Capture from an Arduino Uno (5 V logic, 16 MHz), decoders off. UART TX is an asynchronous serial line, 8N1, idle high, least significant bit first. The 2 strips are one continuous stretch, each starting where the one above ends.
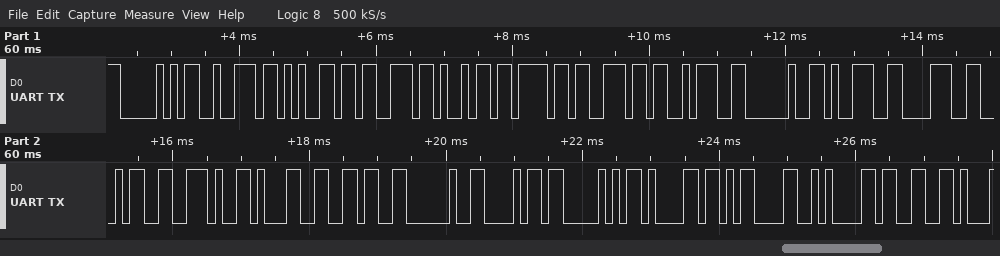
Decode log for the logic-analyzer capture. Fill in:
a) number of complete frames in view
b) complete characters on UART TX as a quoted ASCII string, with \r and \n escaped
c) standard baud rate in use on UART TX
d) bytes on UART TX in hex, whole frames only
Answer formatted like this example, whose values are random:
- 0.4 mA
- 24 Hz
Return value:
- 22
- "Presion: 984.16 hPa\r\n3"
- 9600 baud
- 50 72 65 73 69 6F 6E 3A 20 39 38 34 2E 31 36 20 68 50 61 0D 0A 33
